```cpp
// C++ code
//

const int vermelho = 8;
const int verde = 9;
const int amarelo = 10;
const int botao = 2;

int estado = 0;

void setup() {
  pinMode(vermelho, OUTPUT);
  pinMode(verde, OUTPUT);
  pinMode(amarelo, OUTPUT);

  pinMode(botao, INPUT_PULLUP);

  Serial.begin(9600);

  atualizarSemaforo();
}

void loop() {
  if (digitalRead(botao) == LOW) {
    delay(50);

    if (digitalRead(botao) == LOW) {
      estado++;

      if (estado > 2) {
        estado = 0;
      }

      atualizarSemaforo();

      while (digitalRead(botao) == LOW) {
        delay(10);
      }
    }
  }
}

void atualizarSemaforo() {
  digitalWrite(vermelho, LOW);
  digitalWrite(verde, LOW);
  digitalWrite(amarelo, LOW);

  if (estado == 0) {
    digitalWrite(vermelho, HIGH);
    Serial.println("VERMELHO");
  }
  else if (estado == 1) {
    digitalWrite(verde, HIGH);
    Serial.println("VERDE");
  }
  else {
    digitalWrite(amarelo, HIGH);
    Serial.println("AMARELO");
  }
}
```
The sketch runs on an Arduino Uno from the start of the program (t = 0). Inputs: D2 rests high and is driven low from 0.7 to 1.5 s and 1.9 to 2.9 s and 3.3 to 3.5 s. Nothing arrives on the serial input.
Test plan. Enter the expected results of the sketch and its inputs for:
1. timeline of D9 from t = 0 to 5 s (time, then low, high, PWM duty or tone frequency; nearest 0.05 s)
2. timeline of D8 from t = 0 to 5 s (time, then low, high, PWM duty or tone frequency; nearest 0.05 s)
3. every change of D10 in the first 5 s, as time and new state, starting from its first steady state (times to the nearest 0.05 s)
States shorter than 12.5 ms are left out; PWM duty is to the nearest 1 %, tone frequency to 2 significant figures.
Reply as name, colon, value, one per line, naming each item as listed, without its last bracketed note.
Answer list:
timeline of D9 from t = 0 to 5 s: 0 s low; 0.75 s high; 1.95 s low
timeline of D8 from t = 0 to 5 s: 0 s high; 0.75 s low; 3.35 s high
every change of D10 in the first 5 s, as time and new state, starting from its first steady state: 0 s low; 1.95 s high; 3.35 s low
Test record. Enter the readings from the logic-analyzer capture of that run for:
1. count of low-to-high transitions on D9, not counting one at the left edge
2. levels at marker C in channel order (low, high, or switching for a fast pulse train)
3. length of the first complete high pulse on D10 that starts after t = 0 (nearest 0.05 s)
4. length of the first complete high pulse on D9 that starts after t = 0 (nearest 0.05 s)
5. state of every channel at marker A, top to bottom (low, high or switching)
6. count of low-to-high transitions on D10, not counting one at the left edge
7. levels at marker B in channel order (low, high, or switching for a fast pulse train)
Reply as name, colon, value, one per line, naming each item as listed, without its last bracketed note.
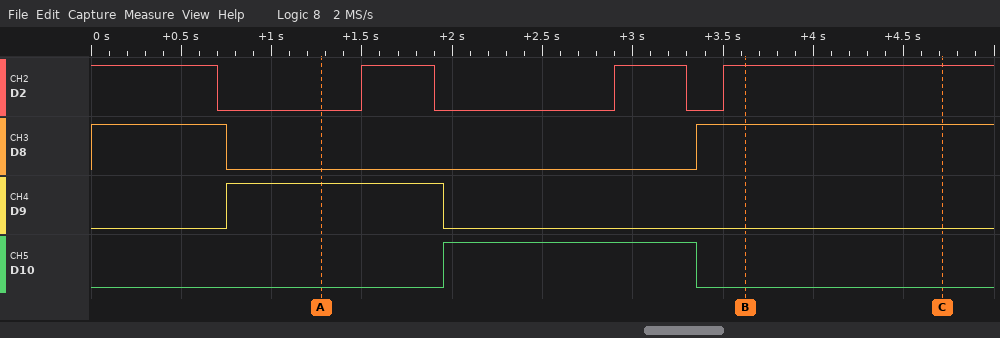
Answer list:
count of low-to-high transitions on D9, not counting one at the left edge: 1
levels at marker C in channel order: D2 high, D8 high, D9 low, D10 low
length of the first complete high pulse on D10 that starts after t = 0: 1.40 s
length of the first complete high pulse on D9 that starts after t = 0: 1.20 s
state of every channel at marker A, top to bottom: D2 low, D8 low, D9 high, D10 low
count of low-to-high transitions on D10, not counting one at the left edge: 1
levels at marker B in channel order: D2 high, D8 high, D9 low, D10 low
